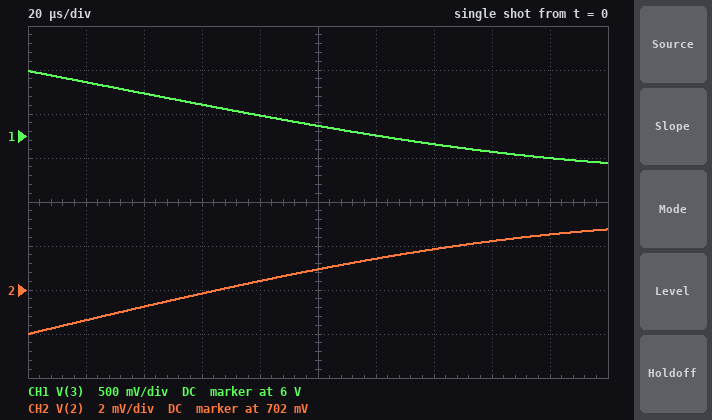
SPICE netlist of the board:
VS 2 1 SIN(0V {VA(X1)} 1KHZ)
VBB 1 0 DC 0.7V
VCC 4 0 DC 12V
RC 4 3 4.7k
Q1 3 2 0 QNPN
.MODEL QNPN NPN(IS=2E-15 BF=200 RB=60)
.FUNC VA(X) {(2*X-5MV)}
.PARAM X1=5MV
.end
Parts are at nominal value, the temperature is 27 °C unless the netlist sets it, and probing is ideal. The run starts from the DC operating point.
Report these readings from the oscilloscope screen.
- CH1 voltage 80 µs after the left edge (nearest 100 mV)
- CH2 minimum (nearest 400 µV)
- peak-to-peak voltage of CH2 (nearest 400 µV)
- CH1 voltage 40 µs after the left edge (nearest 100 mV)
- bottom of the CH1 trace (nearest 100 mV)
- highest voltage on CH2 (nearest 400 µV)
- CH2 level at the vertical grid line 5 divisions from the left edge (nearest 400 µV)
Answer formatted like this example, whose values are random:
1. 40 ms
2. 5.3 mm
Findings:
1. 6.2 V
2. 700.0 mV
3. 4.8 mV
4. 6.5 V
5. 5.7 V
6. 704.8 mV
7. 702.8 mV
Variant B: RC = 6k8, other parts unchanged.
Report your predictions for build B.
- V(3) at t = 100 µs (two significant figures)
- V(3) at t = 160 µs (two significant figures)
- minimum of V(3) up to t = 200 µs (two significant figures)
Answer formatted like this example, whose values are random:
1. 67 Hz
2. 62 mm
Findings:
1. 3.5 V
2. 3.1 V
3. 2.9 V
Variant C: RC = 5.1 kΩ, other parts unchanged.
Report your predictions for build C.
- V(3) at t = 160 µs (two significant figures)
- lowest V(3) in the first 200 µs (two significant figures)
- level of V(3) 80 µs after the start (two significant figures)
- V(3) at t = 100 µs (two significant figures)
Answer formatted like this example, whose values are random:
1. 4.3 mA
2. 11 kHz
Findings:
1. 5.3 V
2. 5.2 V
3. 5.7 V
4. 5.6 V
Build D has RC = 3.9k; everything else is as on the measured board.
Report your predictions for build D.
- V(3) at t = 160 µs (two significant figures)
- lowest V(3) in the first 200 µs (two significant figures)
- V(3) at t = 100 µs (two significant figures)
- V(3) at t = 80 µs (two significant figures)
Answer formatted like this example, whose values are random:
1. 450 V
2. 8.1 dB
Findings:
1. 6.9 V
2. 6.8 V
3. 7.1 V
4. 7.2 V
